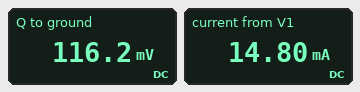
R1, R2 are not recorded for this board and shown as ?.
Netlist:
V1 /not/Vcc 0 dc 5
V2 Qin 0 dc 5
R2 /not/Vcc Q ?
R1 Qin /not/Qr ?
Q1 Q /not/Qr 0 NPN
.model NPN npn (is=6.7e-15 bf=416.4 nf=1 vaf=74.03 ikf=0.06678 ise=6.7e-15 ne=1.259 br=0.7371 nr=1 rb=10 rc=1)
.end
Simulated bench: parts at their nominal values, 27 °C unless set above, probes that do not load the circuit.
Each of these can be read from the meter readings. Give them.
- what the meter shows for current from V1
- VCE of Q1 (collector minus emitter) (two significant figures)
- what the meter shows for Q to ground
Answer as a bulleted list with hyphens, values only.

- 14.80 mA
- 120 mV
- 116.2 mV
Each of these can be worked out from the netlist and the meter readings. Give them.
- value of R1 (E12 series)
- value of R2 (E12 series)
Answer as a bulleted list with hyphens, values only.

- 6.8 kΩ
- 330 Ω
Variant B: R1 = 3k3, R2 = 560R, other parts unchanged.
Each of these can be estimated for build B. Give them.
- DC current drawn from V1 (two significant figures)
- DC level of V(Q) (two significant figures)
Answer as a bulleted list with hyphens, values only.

- 8.8 mA
- 77 mV
